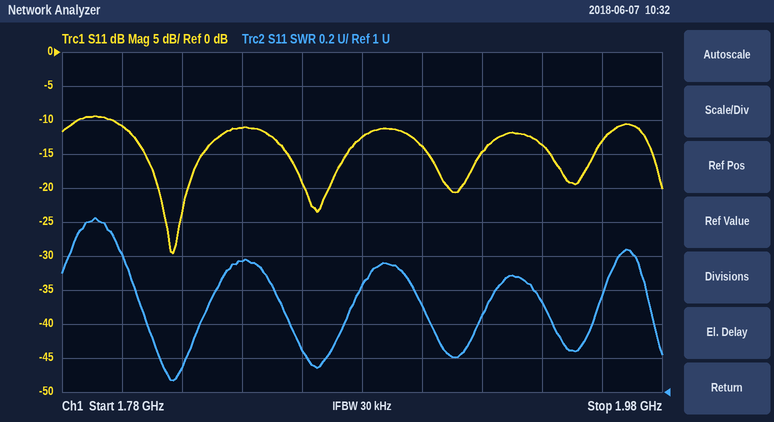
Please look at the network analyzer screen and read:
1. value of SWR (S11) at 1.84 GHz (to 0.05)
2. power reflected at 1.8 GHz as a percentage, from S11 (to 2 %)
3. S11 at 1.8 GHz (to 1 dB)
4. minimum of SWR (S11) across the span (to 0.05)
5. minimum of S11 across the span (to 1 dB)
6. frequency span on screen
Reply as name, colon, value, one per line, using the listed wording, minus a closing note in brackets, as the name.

value of SWR (S11) at 1.84 GHz: 1.75
power reflected at 1.8 GHz as a percentage, from S11: 8 %
S11 at 1.8 GHz: -11 dB
minimum of SWR (S11) across the span: 1.05
minimum of S11 across the span: -30 dB
frequency span on screen: 200 MHz
